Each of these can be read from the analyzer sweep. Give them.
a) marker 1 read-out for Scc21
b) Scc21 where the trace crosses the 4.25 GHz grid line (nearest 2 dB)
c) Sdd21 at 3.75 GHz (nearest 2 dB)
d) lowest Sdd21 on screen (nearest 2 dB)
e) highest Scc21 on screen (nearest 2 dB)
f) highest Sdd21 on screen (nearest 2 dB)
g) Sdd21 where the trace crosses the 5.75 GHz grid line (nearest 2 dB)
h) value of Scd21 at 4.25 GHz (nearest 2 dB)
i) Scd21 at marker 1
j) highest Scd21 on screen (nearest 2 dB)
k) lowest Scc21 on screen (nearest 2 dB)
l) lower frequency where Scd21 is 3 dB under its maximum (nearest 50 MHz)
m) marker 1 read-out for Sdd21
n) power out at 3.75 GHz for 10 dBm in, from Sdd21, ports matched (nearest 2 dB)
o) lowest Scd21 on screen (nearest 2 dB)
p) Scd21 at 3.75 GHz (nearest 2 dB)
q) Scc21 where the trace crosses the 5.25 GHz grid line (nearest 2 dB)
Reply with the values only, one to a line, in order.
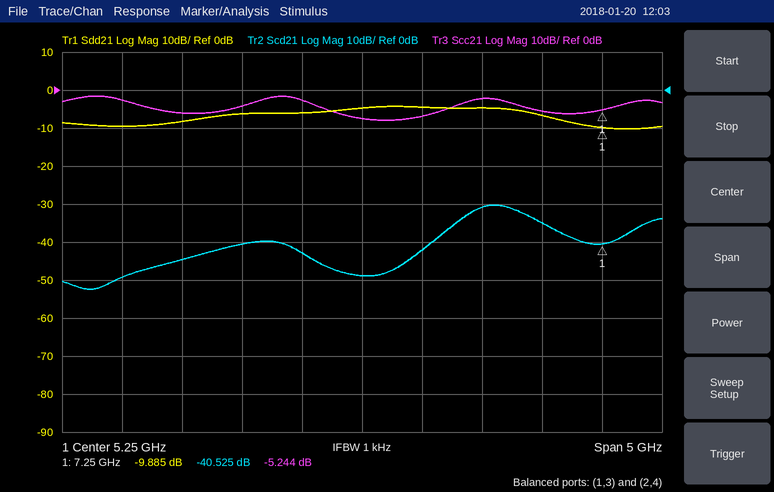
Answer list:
-5.244 dB
-4 dB
-8 dB
-10 dB
-2 dB
-4 dB
-4 dB
-40 dB
-40.525 dB
-30 dB
-8 dB
6.10 GHz
-9.885 dB
2 dBm
-52 dB
-44 dB
-8 dB
